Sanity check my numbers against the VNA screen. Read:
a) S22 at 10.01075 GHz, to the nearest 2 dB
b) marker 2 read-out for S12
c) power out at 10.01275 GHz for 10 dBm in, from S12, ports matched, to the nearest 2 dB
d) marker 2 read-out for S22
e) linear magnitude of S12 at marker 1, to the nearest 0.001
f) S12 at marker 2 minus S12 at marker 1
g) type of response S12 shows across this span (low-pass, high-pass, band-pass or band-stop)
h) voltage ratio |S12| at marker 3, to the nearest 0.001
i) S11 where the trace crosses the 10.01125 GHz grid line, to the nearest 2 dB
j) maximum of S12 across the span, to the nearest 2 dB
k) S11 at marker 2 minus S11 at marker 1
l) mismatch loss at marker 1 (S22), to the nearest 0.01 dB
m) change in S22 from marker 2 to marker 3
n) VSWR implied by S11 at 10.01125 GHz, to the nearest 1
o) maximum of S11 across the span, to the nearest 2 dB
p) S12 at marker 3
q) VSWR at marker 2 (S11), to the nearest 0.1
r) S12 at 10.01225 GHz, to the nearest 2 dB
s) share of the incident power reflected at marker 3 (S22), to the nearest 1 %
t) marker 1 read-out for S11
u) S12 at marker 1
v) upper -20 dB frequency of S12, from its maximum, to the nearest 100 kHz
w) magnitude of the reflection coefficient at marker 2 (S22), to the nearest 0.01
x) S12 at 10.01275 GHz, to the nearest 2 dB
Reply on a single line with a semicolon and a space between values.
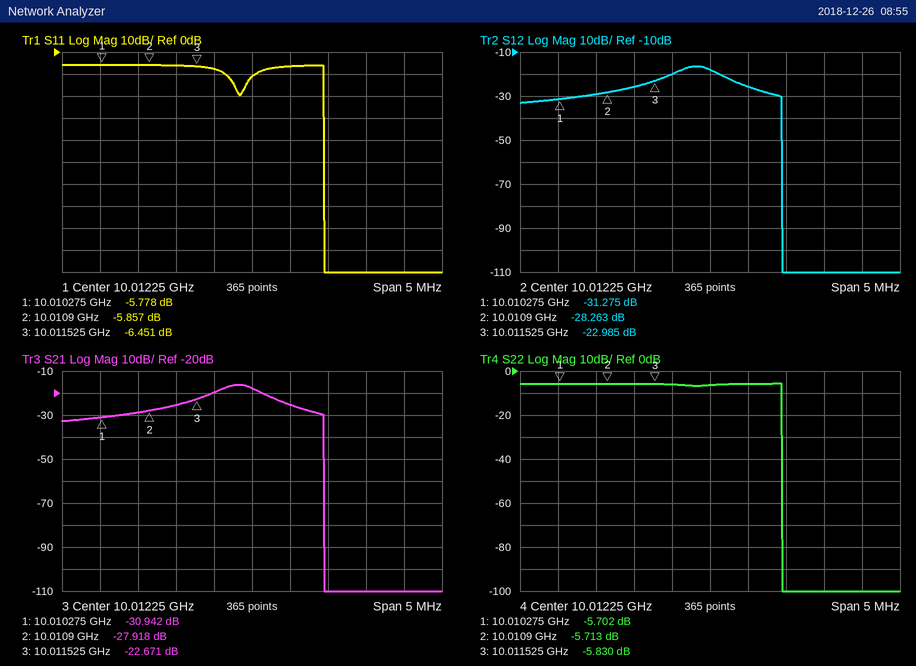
-6 dB; -28.263 dB; -16 dBm; -5.713 dB; 0.027; 3.012 dB; band-pass; 0.071; -6 dB; -16 dB; -0.079 dB; 1.36 dB; -0.117 dB; 3; -6 dB; -22.985 dB; 3.1; -18 dB; 26 %; -5.778 dB; -31.275 dB; 10.0132 GHz; 0.52; -26 dB
